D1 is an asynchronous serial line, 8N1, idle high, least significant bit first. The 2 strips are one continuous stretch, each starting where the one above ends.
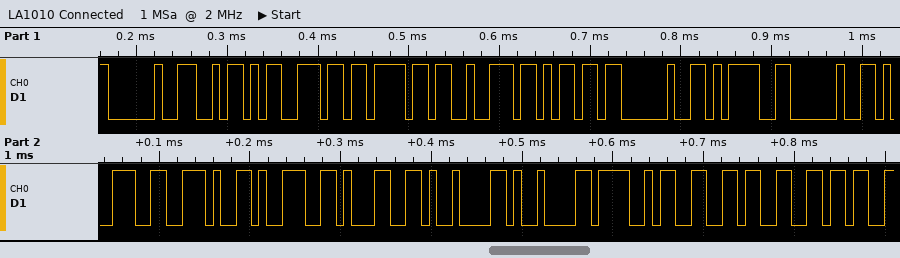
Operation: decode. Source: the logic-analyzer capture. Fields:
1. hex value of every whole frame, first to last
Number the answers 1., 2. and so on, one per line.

1. 0x20 0x5A 0x6E 0x6F 0x72 0x6D 0x20 0x3D 0x20 0x39 0x2E 0x39 0x31 0x09 0x09 0x4F 0x66 0x66
